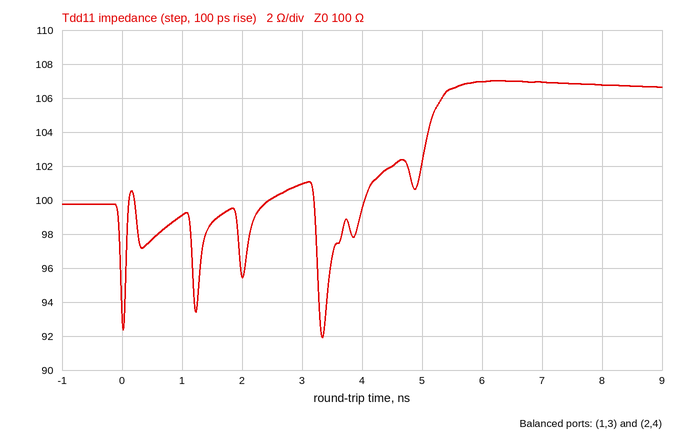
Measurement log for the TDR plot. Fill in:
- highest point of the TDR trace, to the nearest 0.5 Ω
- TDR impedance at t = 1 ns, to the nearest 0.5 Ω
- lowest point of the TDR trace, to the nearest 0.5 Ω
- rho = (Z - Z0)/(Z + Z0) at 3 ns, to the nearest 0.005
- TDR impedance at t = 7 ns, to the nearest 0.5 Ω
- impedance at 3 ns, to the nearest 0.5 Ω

107.0 Ω
99.0 Ω
92.0 Ω
+0.005
107.0 Ω
101.0 Ω
